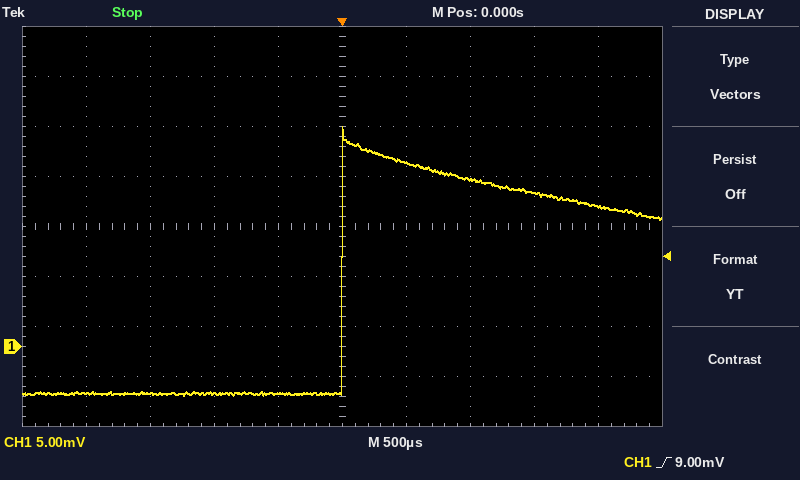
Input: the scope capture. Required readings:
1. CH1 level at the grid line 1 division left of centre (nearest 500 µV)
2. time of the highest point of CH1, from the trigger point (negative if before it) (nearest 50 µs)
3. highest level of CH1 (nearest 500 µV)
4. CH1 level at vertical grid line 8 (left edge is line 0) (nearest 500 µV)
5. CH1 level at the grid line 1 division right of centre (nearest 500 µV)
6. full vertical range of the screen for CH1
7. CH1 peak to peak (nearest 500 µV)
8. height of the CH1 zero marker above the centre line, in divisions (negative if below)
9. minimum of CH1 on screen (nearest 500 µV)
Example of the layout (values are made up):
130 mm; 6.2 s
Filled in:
-4.5 mV; 0 µs; 22.0 mV; 15.5 mV; 18.5 mV; 40 mV; 27.0 mV; -2.4 div; -5.0 mV
